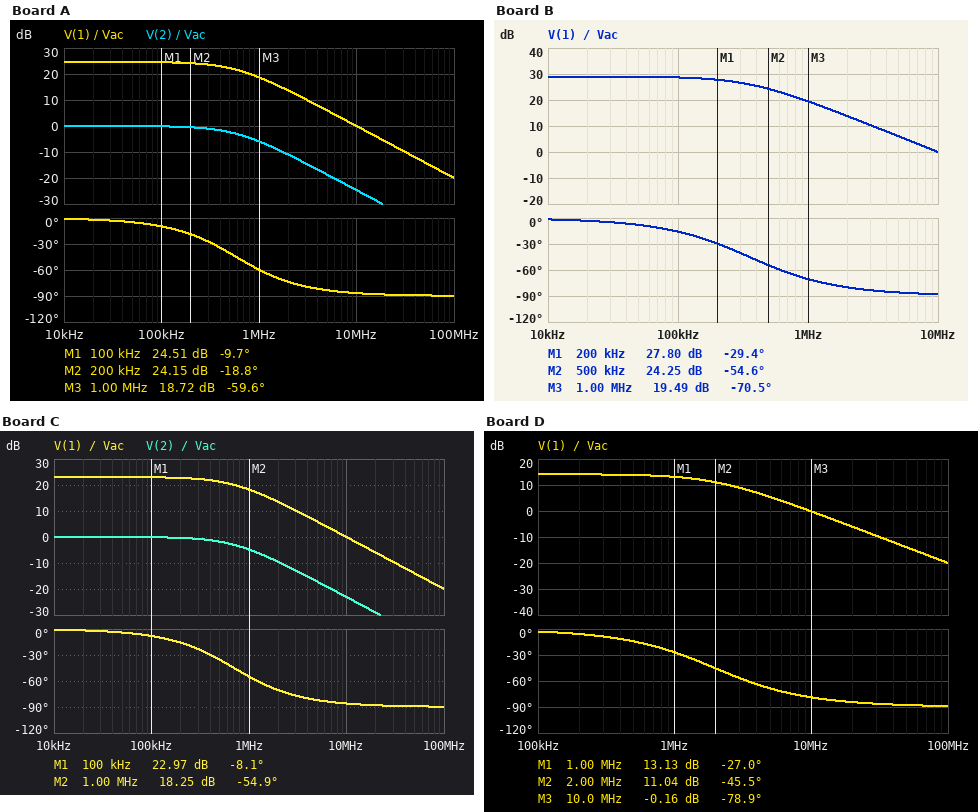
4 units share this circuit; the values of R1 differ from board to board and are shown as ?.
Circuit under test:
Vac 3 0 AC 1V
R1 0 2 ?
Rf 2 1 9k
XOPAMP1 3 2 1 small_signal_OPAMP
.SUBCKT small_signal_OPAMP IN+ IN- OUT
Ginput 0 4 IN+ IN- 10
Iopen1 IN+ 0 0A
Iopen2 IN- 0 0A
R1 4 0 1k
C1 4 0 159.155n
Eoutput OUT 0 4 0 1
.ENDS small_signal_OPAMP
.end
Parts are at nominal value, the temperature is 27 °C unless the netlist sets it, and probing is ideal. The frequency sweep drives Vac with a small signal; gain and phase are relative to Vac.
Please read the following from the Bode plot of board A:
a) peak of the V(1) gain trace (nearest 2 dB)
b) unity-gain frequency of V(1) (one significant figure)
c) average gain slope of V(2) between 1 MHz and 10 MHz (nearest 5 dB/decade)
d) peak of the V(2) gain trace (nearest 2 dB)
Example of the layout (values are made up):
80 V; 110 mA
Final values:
24 dB; 10 MHz; -20 dB/decade; 0 dB
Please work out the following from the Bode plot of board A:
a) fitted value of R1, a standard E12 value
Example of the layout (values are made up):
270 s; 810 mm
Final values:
560 Ω
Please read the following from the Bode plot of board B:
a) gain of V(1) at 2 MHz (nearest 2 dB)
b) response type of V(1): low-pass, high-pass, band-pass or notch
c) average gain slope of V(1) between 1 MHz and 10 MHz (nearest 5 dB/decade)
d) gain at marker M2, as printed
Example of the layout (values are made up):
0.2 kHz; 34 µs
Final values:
14 dB; low-pass; -20 dB/decade; 24.25 dB
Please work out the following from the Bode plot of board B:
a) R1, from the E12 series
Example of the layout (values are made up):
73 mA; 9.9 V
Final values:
330 Ω
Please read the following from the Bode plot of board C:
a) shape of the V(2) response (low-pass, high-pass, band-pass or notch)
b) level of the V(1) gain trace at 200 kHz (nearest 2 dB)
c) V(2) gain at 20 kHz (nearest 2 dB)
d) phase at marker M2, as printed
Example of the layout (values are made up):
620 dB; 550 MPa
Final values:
low-pass; 22 dB; 0 dB; -54.9 deg
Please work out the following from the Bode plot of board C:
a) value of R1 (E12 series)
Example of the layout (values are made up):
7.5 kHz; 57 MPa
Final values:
680 Ω
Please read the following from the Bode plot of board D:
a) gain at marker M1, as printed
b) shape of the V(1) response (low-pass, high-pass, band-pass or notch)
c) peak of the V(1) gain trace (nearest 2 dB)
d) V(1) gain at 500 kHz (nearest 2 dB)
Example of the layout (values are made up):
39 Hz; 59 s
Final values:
13.13 dB; low-pass; 14 dB; 14 dB
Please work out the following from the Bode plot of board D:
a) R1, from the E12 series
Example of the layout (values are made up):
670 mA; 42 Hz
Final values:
2.2 kΩ
